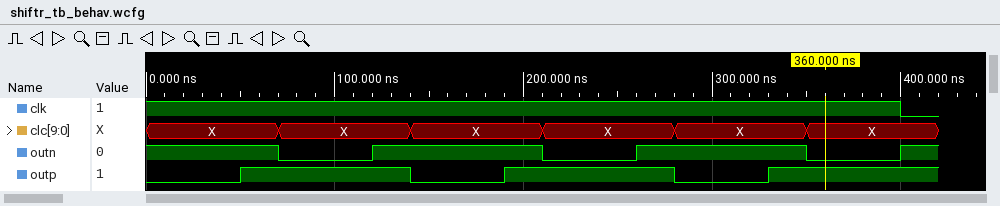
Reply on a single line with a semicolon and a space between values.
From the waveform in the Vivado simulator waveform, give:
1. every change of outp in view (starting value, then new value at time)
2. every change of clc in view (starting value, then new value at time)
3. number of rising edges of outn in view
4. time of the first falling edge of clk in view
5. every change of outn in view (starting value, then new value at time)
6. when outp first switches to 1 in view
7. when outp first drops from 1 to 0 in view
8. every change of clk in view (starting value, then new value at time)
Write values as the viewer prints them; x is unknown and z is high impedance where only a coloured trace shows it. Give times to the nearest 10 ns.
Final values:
0, 1 at 50 ns, 0 at 140 ns, 1 at 190 ns, 0 at 280 ns, 1 at 330 ns; X, X at 70 ns, X at 140 ns, X at 210 ns, X at 280 ns, X at 350 ns; 3; 400 ns; 1, 0 at 70 ns, 1 at 120 ns, 0 at 210 ns, 1 at 260 ns, 0 at 350 ns, 1 at 400 ns; 50 ns; 140 ns; 1, 0 at 400 ns
